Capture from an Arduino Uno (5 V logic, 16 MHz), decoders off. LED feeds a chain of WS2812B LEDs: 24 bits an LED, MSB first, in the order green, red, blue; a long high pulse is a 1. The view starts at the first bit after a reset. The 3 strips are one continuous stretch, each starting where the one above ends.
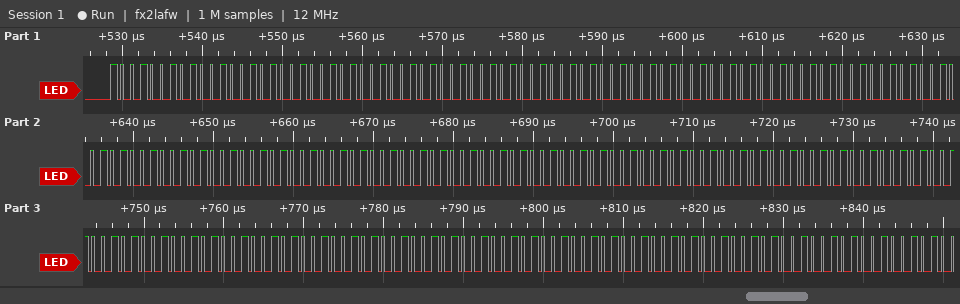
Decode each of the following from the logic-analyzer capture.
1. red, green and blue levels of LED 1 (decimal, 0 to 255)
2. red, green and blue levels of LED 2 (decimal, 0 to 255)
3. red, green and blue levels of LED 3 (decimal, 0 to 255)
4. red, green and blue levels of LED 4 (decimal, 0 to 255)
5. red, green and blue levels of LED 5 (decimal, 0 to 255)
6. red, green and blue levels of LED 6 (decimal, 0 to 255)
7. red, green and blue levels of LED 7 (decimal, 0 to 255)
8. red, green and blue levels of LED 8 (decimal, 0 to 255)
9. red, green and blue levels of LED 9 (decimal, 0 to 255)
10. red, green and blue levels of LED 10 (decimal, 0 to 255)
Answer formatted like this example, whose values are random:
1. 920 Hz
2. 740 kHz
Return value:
1. 146, 146, 146
2. 146, 146, 146
3. 146, 146, 146
4. 146, 146, 146
5. 146, 146, 146
6. 146, 146, 146
7. 146, 146, 146
8. 146, 146, 146
9. 146, 146, 146
10. 146, 146, 146
